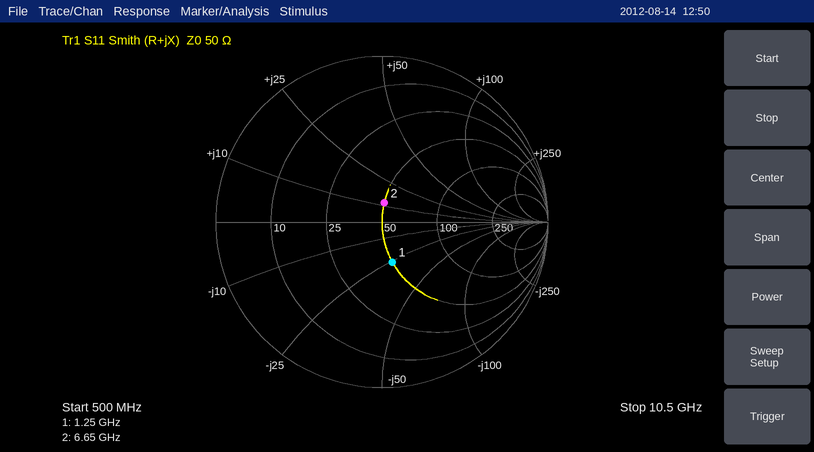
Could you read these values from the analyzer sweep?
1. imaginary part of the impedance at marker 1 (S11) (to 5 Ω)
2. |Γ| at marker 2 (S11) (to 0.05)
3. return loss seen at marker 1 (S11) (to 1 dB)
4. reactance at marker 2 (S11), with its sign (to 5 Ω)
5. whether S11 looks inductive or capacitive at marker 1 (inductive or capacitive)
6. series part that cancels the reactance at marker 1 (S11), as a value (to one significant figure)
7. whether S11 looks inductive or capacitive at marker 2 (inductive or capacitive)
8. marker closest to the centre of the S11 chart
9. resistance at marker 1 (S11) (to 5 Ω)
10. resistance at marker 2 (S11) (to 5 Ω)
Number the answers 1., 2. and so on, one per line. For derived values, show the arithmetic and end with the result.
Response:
1. -25 Ω
2. 0.10
3. 12 dB
4. +10 Ω
5. capacitive
6. L = 25 Ω/(2π × 1.25 GHz) ≈ 3 nH
7. inductive
8. marker 2
9. 50 Ω
10. 50 Ω
